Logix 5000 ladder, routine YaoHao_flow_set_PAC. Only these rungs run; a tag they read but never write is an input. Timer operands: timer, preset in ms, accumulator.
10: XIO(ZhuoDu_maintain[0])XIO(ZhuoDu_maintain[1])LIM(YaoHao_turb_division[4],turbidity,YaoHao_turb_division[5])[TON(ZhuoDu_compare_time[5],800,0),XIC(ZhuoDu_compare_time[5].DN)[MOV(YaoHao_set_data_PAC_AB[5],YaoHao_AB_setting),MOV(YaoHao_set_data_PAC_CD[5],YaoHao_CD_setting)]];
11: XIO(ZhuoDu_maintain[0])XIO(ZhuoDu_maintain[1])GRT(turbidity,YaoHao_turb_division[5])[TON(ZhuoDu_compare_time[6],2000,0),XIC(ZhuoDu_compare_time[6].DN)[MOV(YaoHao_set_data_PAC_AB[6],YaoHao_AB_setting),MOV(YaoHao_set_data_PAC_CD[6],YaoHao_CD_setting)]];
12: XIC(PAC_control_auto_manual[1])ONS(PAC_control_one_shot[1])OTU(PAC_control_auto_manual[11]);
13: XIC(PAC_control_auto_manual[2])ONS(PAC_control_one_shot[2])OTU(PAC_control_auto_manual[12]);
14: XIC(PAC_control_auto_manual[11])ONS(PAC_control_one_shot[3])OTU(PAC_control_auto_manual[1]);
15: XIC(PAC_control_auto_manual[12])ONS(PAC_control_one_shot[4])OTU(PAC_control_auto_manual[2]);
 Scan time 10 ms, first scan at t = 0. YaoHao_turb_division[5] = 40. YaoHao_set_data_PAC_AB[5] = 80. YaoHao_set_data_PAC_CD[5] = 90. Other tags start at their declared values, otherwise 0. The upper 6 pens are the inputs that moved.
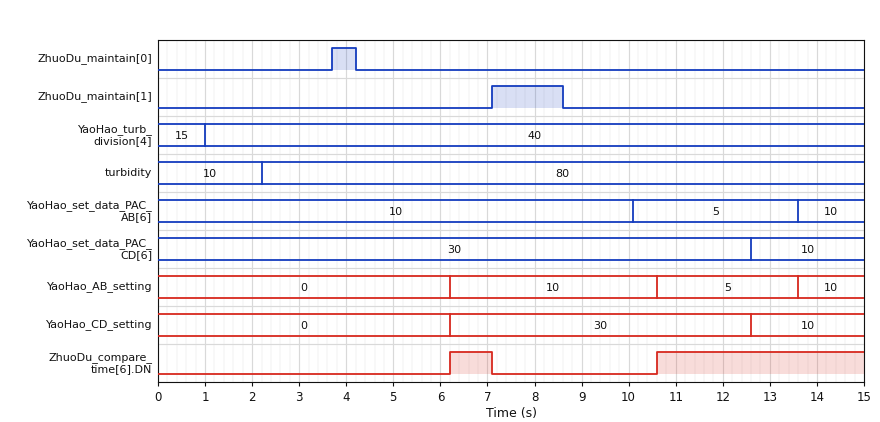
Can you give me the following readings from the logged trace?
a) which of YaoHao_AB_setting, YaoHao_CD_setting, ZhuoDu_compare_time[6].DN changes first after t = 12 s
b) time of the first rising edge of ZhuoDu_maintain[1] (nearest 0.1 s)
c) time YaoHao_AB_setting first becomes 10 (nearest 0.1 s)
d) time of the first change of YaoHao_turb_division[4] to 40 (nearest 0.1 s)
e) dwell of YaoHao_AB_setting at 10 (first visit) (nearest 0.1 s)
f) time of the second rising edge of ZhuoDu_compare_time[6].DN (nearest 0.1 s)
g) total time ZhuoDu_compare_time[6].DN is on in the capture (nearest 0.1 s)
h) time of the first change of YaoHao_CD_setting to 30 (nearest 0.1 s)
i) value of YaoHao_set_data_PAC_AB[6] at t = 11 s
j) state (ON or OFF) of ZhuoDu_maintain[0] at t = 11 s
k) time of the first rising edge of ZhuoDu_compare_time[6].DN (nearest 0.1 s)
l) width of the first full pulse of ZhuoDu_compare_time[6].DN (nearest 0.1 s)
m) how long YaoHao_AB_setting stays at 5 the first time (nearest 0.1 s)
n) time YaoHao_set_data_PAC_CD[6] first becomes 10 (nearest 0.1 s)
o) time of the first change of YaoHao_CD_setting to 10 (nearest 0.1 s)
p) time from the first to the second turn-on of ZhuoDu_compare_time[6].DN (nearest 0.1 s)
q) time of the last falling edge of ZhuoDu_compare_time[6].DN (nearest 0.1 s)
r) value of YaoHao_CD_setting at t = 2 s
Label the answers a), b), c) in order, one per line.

a) YaoHao_CD_setting
b) 7.1 s
c) 6.2 s
d) 1.0 s
e) 4.4 s
f) 10.6 s
g) 5.3 s
h) 6.2 s
i) 5
j) OFF
k) 6.2 s
l) 0.9 s
m) 3.0 s
n) 12.6 s
o) 12.6 s
p) 4.4 s
q) 7.1 s
r) 0
